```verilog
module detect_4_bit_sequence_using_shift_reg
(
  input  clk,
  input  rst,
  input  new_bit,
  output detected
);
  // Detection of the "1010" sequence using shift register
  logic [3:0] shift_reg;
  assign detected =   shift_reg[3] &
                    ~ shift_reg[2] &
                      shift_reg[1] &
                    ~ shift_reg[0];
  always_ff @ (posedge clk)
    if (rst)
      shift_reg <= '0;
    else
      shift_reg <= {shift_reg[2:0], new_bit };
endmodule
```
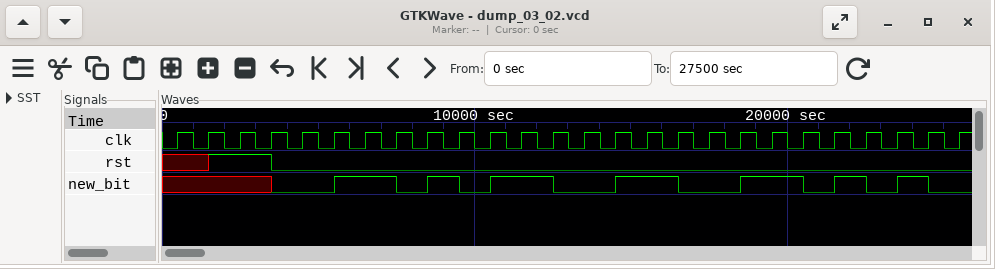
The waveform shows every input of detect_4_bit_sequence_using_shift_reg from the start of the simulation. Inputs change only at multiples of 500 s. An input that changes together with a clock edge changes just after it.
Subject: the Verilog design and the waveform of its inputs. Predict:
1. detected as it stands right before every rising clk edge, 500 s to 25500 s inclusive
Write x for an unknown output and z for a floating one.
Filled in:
x x x 0 0 0 0 0 0 0 0 1 0 0 0 0 0 0 0 0 0 0 0 0 1 0
